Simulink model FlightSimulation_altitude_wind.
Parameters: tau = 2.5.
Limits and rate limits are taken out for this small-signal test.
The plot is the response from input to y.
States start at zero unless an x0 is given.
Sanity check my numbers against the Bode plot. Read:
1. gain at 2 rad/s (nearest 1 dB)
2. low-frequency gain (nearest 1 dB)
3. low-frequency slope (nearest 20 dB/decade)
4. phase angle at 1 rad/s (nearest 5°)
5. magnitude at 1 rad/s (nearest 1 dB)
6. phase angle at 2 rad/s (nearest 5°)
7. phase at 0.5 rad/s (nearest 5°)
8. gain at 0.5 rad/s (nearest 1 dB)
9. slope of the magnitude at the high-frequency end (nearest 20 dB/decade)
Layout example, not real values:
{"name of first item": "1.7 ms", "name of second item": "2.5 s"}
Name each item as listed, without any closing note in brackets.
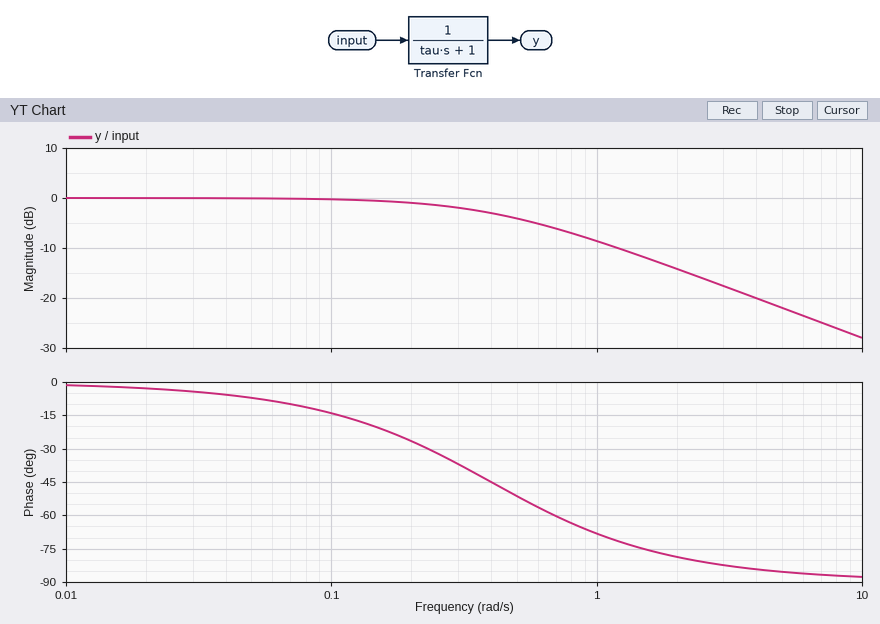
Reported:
{"gain at 2 rad/s": "-14 dB", "low-frequency gain": "0 dB", "low-frequency slope": "0 dB/decade", "phase angle at 1 rad/s": "-70°", "magnitude at 1 rad/s": "-9 dB", "phase angle at 2 rad/s": "-80°", "phase at 0.5 rad/s": "-50°", "gain at 0.5 rad/s": "-4 dB", "slope of the magnitude at the high-frequency end": "-20 dB/decade"}
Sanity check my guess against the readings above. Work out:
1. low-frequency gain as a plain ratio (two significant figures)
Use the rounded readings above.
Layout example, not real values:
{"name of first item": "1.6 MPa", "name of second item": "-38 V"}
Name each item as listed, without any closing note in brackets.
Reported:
{"low-frequency gain as a plain ratio": "1.0"}
